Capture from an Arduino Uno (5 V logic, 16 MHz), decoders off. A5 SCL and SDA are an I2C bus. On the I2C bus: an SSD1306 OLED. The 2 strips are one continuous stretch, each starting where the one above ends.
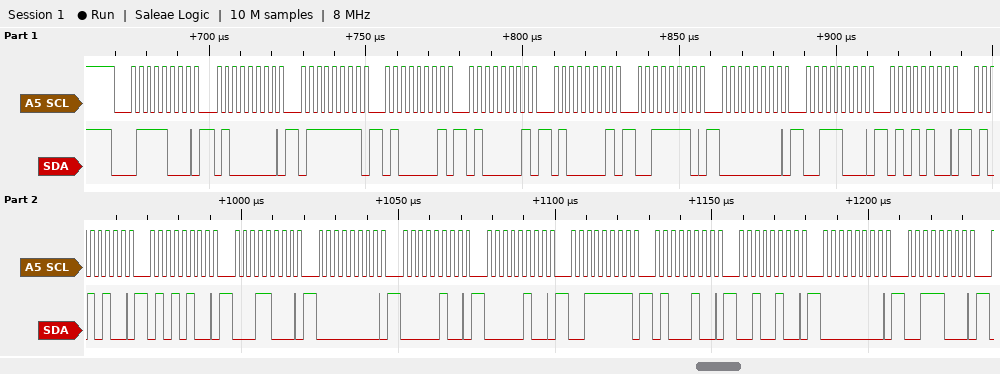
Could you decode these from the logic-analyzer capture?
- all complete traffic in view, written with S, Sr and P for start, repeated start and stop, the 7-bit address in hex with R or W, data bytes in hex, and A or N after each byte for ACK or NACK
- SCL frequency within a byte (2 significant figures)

S 3CW A 40 A 7F A 41 A 41 A 41 A 3E A 00 A 38 A 54 A 54 A 54 A 18 A 00 A 04 A 04 A 3F A 44 A 24 A 00 A 38 A
400 kHz
